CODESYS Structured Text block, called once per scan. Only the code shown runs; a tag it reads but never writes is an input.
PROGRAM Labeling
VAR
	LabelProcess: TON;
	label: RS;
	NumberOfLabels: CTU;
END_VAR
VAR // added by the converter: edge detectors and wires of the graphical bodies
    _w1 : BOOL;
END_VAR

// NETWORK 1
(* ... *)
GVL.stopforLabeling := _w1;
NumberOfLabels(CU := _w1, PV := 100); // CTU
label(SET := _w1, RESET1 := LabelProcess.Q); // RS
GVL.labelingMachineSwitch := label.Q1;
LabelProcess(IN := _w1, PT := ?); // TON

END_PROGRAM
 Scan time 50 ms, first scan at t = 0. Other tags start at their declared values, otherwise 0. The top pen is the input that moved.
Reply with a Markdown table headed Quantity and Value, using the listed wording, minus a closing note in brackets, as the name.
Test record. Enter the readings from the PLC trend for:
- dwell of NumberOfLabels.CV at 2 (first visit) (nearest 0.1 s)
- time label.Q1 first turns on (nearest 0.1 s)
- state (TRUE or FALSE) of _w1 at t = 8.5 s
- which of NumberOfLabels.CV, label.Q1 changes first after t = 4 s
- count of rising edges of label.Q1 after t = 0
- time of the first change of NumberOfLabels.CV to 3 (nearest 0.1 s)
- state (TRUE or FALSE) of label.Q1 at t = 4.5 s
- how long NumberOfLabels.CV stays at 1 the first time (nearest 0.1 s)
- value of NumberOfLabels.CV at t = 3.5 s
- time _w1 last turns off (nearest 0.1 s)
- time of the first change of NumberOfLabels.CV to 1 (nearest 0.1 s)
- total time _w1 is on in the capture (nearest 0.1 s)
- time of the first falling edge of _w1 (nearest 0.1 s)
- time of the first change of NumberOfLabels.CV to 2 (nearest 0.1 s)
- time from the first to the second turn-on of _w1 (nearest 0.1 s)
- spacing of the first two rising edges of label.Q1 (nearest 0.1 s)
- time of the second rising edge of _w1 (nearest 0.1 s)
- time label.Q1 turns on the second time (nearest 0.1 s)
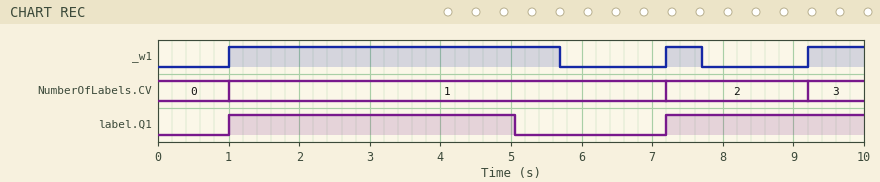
| Quantity | Value |
|---|---|
| dwell of NumberOfLabels.CV at 2 (first visit) | 2.0 s |
| time label.Q1 first turns on | 1.0 s |
| state (TRUE or FALSE) of _w1 at t = 8.5 s | FALSE |
| which of NumberOfLabels.CV, label.Q1 changes first after t = 4 s | label.Q1 |
| count of rising edges of label.Q1 after t = 0 | 2 |
| time of the first change of NumberOfLabels.CV to 3 | 9.2 s |
| state (TRUE or FALSE) of label.Q1 at t = 4.5 s | TRUE |
| how long NumberOfLabels.CV stays at 1 the first time | 6.2 s |
| value of NumberOfLabels.CV at t = 3.5 s | 1 |
| time _w1 last turns off | 7.7 s |
| time of the first change of NumberOfLabels.CV to 1 | 1.0 s |
| total time _w1 is on in the capture | 6.0 s |
| time of the first falling edge of _w1 | 5.7 s |
| time of the first change of NumberOfLabels.CV to 2 | 7.2 s |
| time from the first to the second turn-on of _w1 | 6.2 s |
| spacing of the first two rising edges of label.Q1 | 6.2 s |
| time of the second rising edge of _w1 | 7.2 s |
| time label.Q1 turns on the second time | 7.2 s |
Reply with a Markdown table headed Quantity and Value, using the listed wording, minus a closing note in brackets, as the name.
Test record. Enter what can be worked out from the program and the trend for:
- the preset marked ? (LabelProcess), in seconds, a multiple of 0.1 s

| Quantity | Value |
|---|---|
| the preset marked ? (LabelProcess), in seconds, a multiple of 0.1 s | 4.0 s |
